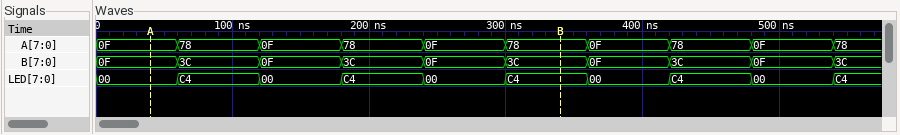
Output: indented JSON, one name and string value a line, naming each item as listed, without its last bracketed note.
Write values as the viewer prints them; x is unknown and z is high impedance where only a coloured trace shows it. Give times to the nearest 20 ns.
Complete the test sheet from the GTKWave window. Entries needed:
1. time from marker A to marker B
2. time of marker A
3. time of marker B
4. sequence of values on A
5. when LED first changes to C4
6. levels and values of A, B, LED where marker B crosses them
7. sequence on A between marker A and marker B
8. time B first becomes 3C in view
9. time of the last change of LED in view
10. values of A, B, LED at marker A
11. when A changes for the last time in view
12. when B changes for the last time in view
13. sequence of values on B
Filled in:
{
  "time from marker A to marker B": "300 ns",
  "time of marker A": "40 ns",
  "time of marker B": "340 ns",
  "sequence of values on A": "0F, 78, 0F, 78, 0F, 78, 0F, 78, 0F, 78",
  "when LED first changes to C4": "60 ns",
  "levels and values of A, B, LED where marker B crosses them": "A=78, B=3C, LED=C4",
  "sequence on A between marker A and marker B": "0F, 78, 0F, 78, 0F, 78",
  "time B first becomes 3C in view": "60 ns",
  "time of the last change of LED in view": "540 ns",
  "values of A, B, LED at marker A": "A=0F, B=0F, LED=00",
  "when A changes for the last time in view": "540 ns",
  "when B changes for the last time in view": "540 ns",
  "sequence of values on B": "0F, 3C, 0F, 3C, 0F, 3C, 0F, 3C, 0F, 3C"
}
